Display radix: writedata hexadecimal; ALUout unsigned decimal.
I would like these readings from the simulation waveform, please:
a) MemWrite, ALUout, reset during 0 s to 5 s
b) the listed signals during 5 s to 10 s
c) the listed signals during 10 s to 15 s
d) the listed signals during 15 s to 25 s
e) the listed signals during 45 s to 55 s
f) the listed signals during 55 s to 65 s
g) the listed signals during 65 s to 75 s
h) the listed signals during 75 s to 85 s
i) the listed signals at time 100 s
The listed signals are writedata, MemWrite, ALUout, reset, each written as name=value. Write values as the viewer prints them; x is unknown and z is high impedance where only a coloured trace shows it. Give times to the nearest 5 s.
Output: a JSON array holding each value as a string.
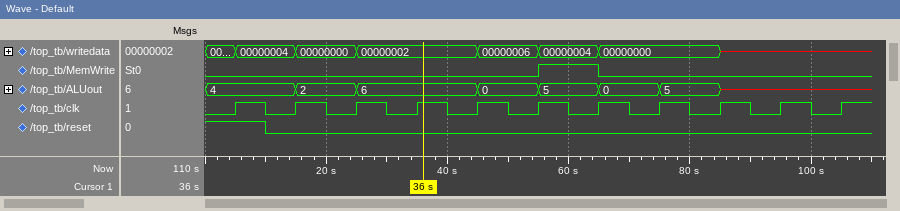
["MemWrite=0, ALUout=4, reset=1", "writedata=00000004, MemWrite=0, ALUout=4, reset=1", "writedata=00000004, MemWrite=0, ALUout=4, reset=0", "writedata=00000000, MemWrite=0, ALUout=2, reset=0", "writedata=00000006, MemWrite=0, ALUout=0, reset=0", "writedata=00000004, MemWrite=1, ALUout=5, reset=0", "writedata=00000000, MemWrite=0, ALUout=0, reset=0", "writedata=00000000, MemWrite=0, ALUout=5, reset=0", "writedata=x, MemWrite=0, ALUout=x, reset=0"]
